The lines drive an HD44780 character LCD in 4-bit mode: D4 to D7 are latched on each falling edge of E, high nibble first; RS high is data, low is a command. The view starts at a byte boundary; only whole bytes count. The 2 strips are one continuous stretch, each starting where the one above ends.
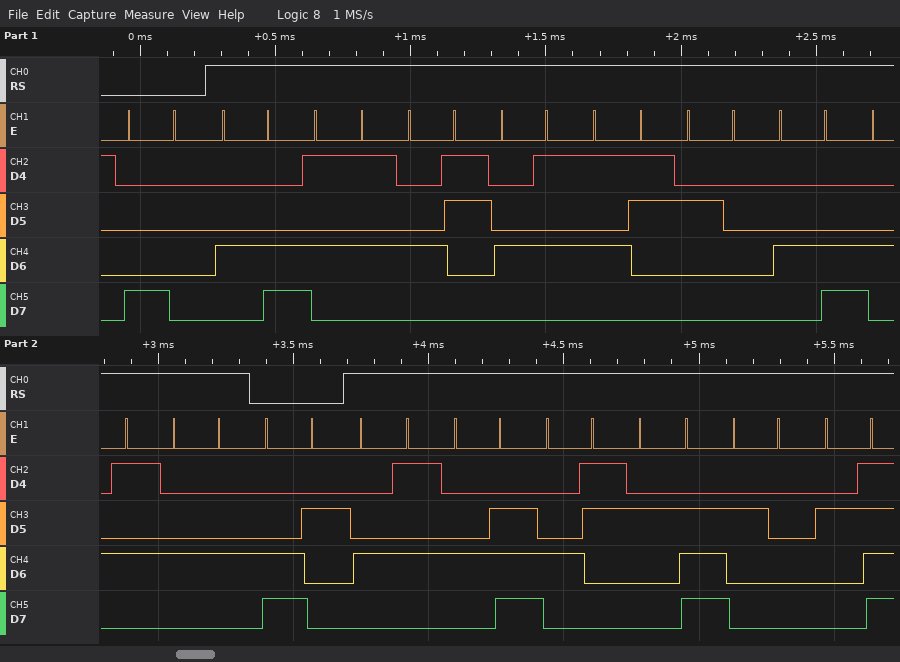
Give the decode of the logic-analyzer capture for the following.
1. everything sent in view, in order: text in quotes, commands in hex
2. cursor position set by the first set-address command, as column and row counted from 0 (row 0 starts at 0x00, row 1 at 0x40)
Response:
0x80 "LUCES LED" 0xC2 "ENC. /"
column 0, row 0
